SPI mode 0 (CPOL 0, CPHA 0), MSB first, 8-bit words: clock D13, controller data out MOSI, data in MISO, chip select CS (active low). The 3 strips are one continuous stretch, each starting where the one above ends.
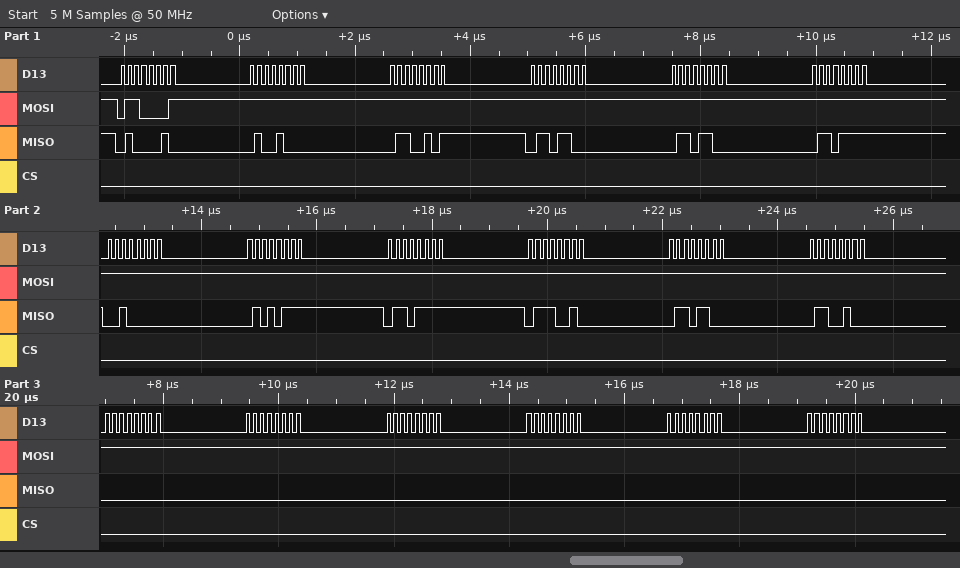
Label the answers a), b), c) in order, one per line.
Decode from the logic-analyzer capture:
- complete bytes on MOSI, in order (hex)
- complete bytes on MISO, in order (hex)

a) 0x61 0xFF 0xFF 0xFF 0xFF 0xFF 0xFF 0xFF 0xFF 0xFF 0xFF 0xFF 0xFF 0xFF 0xFF 0xFF 0xFF 0xFF
b) 0x42 0x48 0x65 0x6C 0x6C 0x6F 0x20 0x57 0x6F 0x72 0x6C 0x64 0x00 0x00 0x00 0x00 0x00 0x00
